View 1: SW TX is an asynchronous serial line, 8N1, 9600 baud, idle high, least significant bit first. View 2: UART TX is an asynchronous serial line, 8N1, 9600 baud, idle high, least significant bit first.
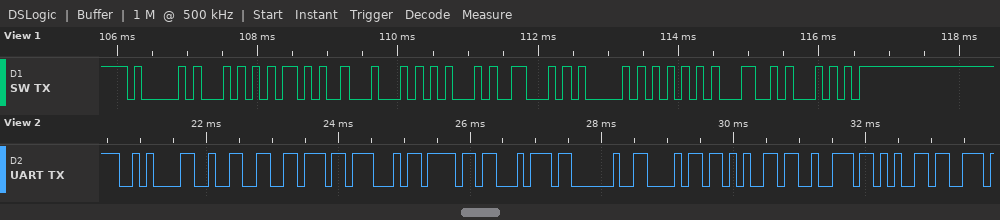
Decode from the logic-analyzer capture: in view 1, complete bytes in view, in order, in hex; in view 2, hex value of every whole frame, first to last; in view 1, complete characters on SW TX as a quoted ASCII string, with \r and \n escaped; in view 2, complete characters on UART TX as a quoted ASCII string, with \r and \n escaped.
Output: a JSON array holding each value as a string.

["41 54 2B 44 45 46 41 55 4C 54", "0x0A 0x32 0x76 0x47 0x6F 0x74 0x20 0x68 0x65 0x72 0x65", "\"AT+DEFAULT\"", "\"\\n2vGot here\""]
